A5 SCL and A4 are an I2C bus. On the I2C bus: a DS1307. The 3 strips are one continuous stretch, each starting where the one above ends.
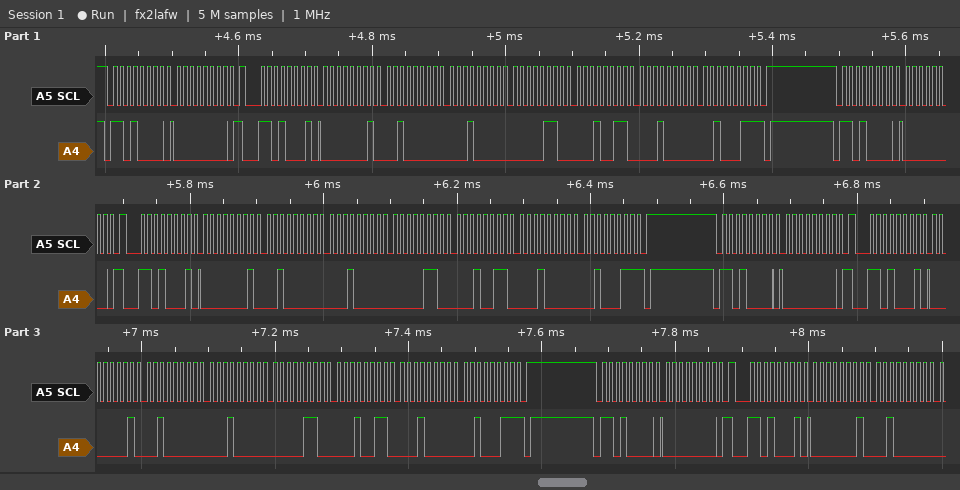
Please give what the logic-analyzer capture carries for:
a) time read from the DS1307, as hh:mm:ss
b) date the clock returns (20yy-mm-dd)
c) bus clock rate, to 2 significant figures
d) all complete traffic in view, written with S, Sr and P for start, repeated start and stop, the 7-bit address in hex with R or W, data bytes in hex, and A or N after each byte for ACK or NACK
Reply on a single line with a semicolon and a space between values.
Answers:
10:20:01; 2023-10-13; 100 kHz; S 68W A 00 A Sr 68R A 01 A 20 A 10 A 06 A 13 A 10 A 23 N P S 68W A 00 A Sr 68R A 01 A 20 A 10 A 06 A 13 A 10 A 23 N P S 68W A 00 A Sr 68R A 01 A 20 A 10 A 06 A 13 A 10 A 23 N P S 68W A 00 A Sr 68R A 01 A 20 A
